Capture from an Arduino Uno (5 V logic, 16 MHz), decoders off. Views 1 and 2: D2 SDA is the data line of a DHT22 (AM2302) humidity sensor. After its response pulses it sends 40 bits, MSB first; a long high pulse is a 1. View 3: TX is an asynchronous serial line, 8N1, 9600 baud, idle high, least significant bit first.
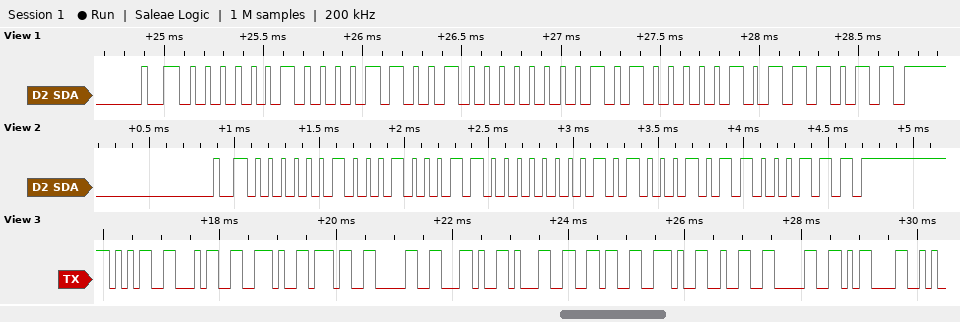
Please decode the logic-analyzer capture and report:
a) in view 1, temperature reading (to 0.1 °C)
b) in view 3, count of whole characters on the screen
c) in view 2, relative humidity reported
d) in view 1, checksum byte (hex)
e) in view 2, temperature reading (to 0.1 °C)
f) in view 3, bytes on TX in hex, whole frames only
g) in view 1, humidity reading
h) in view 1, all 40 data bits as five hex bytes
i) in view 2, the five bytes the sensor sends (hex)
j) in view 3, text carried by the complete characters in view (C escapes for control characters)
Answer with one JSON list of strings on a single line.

["16.0 °C", "12", "54.7 %", "0xBB", "16.2 °C", "35 34 2E 37 30 2C 31 36 2E 32 30 0D", "53.7 %", "02 19 00 A0 BB", "02 23 00 A2 C7", "\"54.70,16.20\\r\""]
